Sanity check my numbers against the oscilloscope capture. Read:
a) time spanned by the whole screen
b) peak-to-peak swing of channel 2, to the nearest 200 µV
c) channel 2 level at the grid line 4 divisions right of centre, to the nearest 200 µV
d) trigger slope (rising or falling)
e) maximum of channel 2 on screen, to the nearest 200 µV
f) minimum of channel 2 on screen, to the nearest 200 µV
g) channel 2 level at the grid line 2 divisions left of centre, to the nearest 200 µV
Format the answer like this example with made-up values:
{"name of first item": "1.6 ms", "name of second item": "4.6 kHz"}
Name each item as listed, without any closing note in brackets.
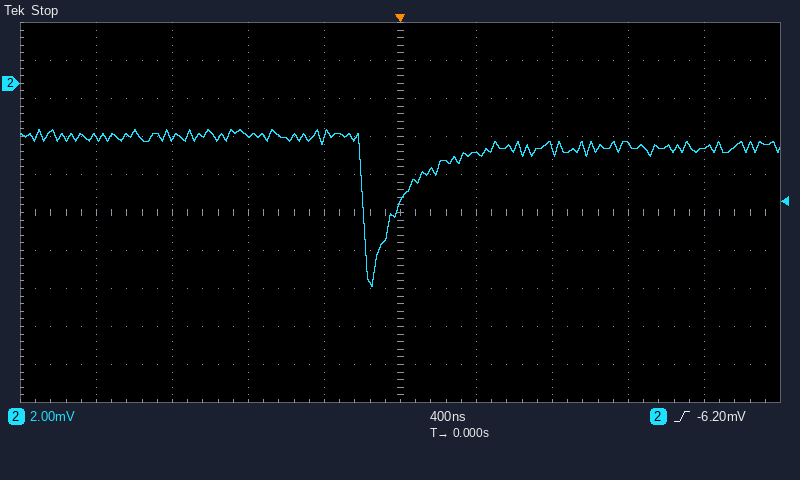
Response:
{"time spanned by the whole screen": "4 µs", "peak-to-peak swing of channel 2, to the nearest 200 µV": "8.2 mV", "channel 2 level at the grid line 4 divisions right of centre, to the nearest 200 µV": "-3.4 mV", "trigger slope": "rising", "maximum of channel 2 on screen, to the nearest 200 µV": "-2.4 mV", "minimum of channel 2 on screen, to the nearest 200 µV": "-10.6 mV", "channel 2 level at the grid line 2 divisions left of centre, to the nearest 200 µV": "-2.8 mV"}
